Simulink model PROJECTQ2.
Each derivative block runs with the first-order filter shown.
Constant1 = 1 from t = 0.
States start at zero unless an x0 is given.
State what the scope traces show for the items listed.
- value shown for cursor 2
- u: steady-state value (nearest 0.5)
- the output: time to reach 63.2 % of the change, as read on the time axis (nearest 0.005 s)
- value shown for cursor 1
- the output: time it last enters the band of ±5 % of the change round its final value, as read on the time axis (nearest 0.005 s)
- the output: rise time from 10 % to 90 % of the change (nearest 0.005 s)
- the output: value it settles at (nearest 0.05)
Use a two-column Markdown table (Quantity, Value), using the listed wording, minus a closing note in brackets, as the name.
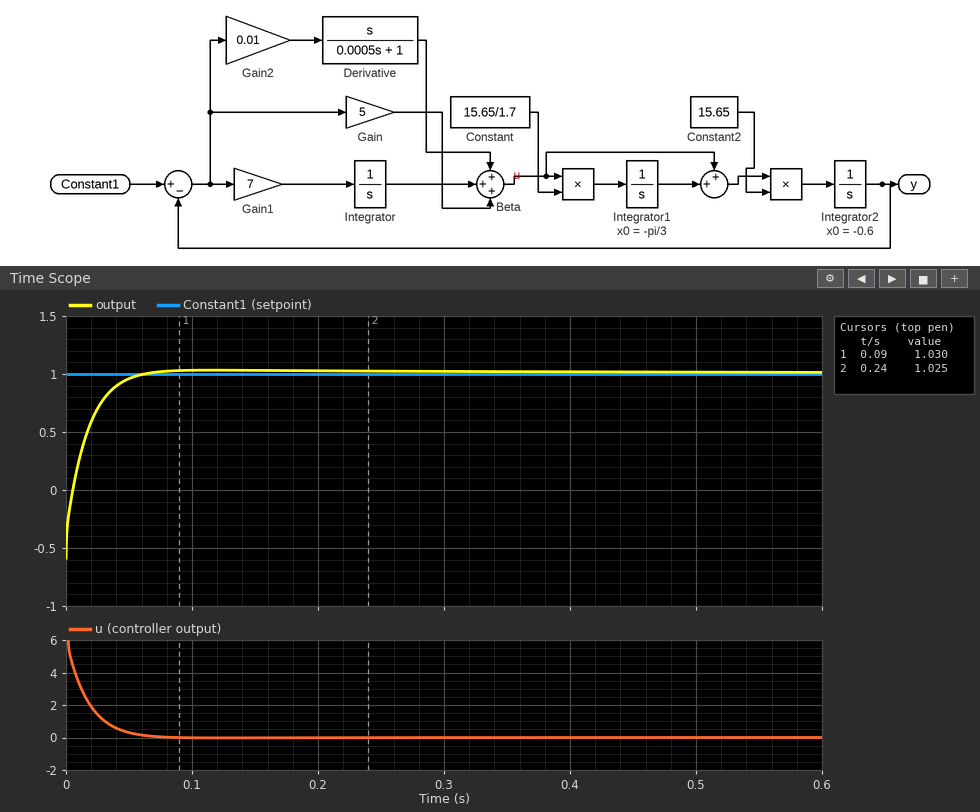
| Quantity | Value |
|---|---|
| value shown for cursor 2 | 1.025 |
| u: steady-state value | 0.0 |
| the output: time to reach 63.2 % of the change, as read on the time axis | 0.015 s |
| value shown for cursor 1 | 1.030 |
| the output: time it last enters the band of ±5 % of the change round its final value, as read on the time axis | 0.045 s |
| the output: rise time from 10 % to 90 % of the change | 0.035 s |
| the output: value it settles at | 1.00 |
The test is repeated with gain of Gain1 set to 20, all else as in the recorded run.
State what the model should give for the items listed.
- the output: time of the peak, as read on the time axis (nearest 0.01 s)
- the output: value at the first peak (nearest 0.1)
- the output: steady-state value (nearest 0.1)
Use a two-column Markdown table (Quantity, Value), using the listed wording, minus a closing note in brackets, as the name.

| Quantity | Value |
|---|---|
| the output: time of the peak, as read on the time axis | 0.09 s |
| the output: value at the first peak | 1.1 |
| the output: steady-state value | 1.0 |
